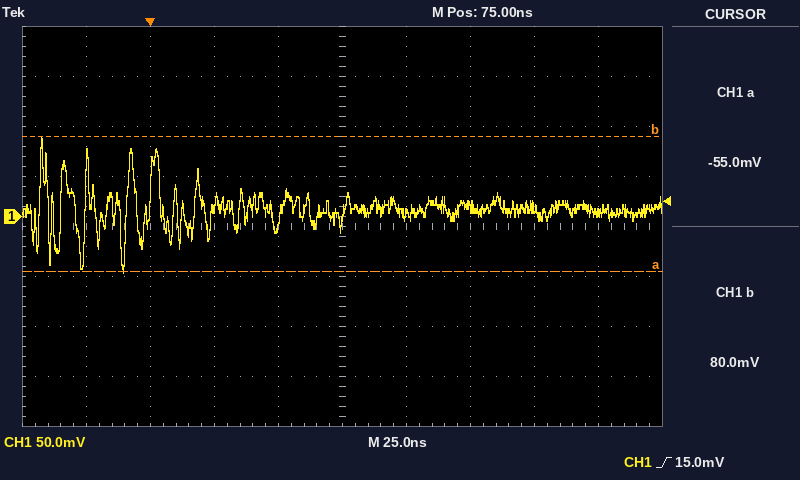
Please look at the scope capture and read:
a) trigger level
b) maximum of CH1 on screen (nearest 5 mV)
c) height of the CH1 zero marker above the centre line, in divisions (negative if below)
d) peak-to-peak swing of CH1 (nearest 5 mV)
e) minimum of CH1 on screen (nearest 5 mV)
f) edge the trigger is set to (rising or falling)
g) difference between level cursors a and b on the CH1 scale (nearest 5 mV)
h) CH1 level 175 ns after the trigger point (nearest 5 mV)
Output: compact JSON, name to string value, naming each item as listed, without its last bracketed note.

{"trigger level": "15.0 mV", "maximum of CH1 on screen": "80 mV", "height of the CH1 zero marker above the centre line, in divisions": "+0.2 div", "peak-to-peak swing of CH1": "135 mV", "minimum of CH1 on screen": "-55 mV", "edge the trigger is set to": "rising", "difference between level cursors a and b on the CH1 scale": "135 mV", "CH1 level 175 ns after the trigger point": "5 mV"}
